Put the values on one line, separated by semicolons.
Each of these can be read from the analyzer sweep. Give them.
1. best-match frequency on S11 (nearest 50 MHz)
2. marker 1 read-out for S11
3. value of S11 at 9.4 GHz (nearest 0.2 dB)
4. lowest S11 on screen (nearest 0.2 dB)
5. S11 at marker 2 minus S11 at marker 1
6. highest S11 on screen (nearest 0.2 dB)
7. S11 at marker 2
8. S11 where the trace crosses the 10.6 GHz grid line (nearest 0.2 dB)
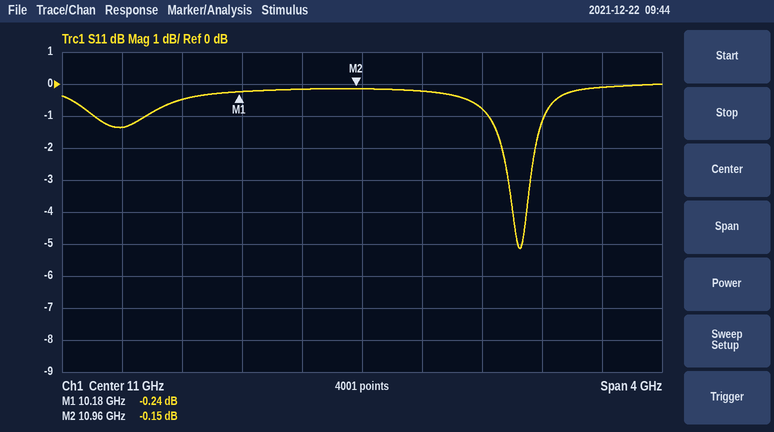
12.05 GHz; -0.24 dB; -1.4 dB; -5.2 dB; 0.09 dB; 0.0 dB; -0.15 dB; -0.2 dB
